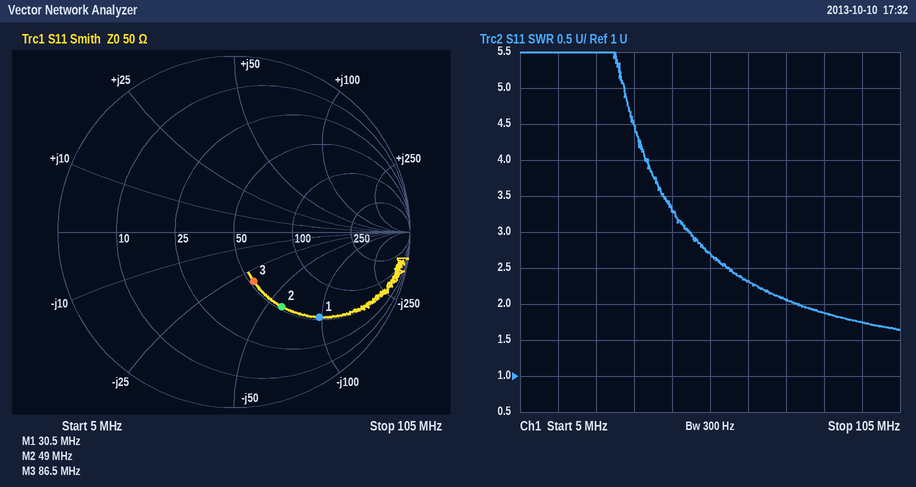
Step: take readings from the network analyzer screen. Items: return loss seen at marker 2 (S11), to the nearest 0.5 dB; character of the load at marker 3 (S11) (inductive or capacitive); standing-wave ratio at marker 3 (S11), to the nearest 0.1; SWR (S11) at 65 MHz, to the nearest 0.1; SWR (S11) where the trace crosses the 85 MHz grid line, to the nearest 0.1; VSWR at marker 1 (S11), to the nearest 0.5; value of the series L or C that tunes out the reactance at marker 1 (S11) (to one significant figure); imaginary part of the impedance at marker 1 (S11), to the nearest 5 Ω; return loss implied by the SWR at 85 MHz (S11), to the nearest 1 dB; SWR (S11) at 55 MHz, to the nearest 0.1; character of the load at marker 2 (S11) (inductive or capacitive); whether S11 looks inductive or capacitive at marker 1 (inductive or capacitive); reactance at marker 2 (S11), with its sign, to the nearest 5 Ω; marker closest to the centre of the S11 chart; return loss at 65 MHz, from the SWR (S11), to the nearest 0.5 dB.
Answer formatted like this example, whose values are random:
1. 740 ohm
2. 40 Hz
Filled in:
1. 6.0 dB
2. capacitive
3. 1.9
4. 2.3
5. 1.9
6. 5.5
7. 500 nH
8. -95 Ω
9. 10 dB
10. 2.7
11. capacitive
12. capacitive
13. -60 Ω
14. marker 3
15. 8.0 dB
